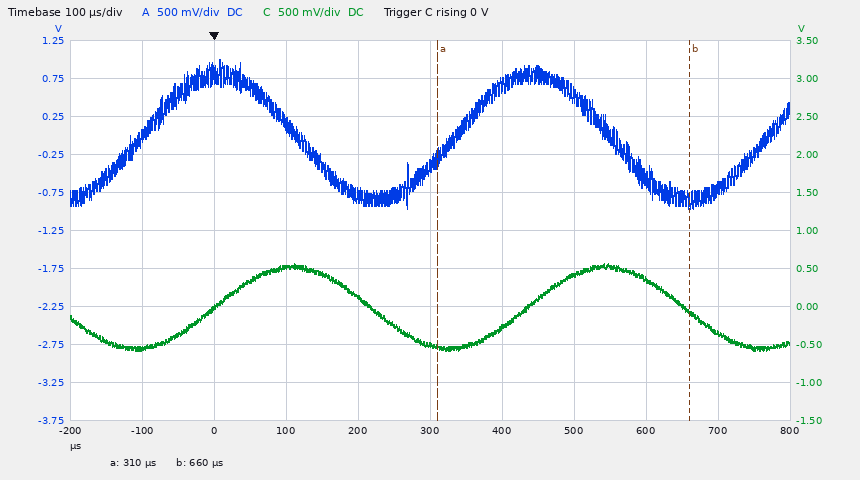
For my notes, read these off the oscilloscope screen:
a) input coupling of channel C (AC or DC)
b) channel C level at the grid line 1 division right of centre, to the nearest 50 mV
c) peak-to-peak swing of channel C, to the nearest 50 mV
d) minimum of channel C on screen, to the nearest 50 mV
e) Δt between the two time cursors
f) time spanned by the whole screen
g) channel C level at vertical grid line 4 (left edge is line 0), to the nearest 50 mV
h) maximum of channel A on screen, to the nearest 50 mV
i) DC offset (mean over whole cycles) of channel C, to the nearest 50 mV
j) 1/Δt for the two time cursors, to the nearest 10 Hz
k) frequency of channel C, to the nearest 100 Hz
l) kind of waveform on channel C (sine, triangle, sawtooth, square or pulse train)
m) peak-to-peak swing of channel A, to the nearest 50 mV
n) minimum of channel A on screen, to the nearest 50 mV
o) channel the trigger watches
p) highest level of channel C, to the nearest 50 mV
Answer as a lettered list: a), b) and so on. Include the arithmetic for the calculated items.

a) DC
b) -300 mV
c) 550 mV − (-600 mV) = 1.15 V
d) -600 mV
e) 660 µs − (310 µs) = 350 µs
f) 1 ms
g) 100 mV
h) 1.00 V
i) (550 mV + (-600 mV)) / 2 ≈ 0 mV
j) 1 / 350 µs ≈ 2.86 kHz
k) 2.3 kHz
l) sine
m) 1.00 V − (-950 mV) = 1.95 V
n) -950 mV
o) channel C
p) 550 mV
